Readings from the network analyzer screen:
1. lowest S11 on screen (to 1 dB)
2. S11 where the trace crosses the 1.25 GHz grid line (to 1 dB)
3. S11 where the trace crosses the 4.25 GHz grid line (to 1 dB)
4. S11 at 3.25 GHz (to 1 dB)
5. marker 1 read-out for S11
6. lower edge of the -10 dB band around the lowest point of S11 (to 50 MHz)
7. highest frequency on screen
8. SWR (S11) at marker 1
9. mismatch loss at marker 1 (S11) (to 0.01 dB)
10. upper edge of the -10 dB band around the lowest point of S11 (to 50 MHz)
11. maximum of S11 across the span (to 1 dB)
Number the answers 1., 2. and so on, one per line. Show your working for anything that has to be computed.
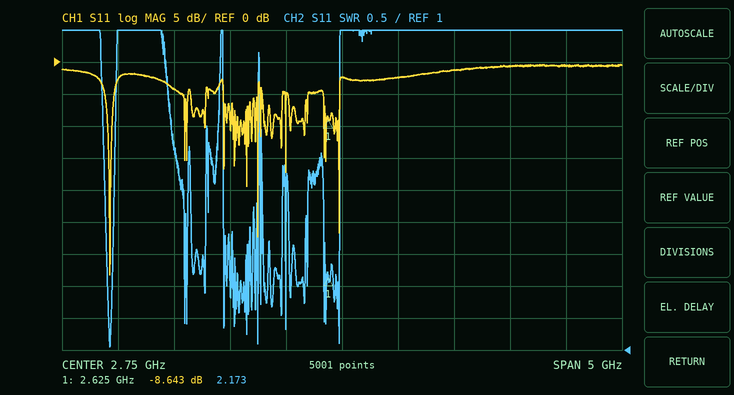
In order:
1. -33 dB
2. -4 dB
3. -1 dB
4. -2 dB
5. -8.643 dB
6. 650 MHz
7. 5.25 GHz
8. 2.173
9. −10 log10(1 − 10^(-8.643/10)) ≈ 0.64 dB
10. 700 MHz
11. 0 dB
